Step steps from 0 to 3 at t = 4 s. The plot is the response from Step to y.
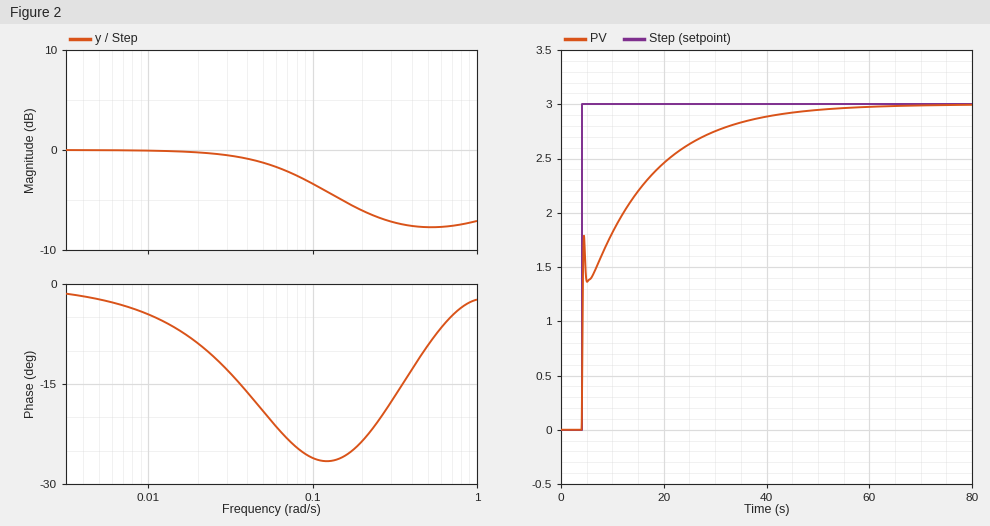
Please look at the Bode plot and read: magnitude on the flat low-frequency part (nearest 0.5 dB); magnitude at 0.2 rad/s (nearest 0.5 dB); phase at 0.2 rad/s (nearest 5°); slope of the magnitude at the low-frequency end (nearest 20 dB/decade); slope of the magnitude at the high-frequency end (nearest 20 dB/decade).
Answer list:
0.0 dB
-6.0 dB
-25°
0 dB/decade
0 dB/decade
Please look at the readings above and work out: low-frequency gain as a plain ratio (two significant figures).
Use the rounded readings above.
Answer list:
1.0
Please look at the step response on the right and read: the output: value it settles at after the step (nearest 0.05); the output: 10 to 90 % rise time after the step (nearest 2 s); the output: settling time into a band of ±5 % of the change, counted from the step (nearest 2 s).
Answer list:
3.00
24 s
32 s
